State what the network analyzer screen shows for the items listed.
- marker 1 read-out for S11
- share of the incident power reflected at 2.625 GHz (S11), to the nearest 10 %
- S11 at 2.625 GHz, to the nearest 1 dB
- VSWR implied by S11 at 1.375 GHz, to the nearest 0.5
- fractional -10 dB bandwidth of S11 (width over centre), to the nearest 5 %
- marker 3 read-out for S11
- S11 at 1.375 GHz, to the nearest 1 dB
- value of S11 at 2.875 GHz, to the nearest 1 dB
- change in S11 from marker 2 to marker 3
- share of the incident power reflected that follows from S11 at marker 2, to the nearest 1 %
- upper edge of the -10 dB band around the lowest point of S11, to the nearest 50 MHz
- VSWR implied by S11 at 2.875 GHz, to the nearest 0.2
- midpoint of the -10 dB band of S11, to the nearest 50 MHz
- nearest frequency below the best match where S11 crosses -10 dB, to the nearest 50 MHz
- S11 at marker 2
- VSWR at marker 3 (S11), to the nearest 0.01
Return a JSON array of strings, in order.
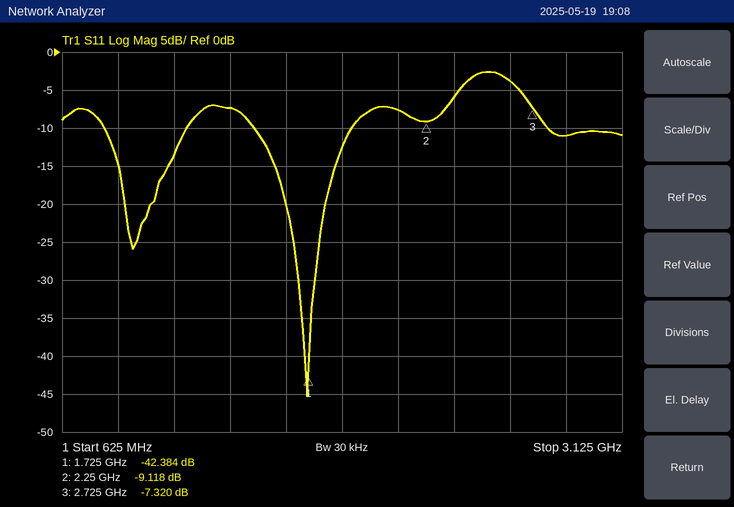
["-42.384 dB", "40 %", "-4 dB", "2.5", "25 %", "-7.320 dB", "-7 dB", "-11 dB", "1.798 dB", "12 %", "1.90 GHz", "1.8", "1.70 GHz", "1.50 GHz", "-9.118 dB", "2.51"]
